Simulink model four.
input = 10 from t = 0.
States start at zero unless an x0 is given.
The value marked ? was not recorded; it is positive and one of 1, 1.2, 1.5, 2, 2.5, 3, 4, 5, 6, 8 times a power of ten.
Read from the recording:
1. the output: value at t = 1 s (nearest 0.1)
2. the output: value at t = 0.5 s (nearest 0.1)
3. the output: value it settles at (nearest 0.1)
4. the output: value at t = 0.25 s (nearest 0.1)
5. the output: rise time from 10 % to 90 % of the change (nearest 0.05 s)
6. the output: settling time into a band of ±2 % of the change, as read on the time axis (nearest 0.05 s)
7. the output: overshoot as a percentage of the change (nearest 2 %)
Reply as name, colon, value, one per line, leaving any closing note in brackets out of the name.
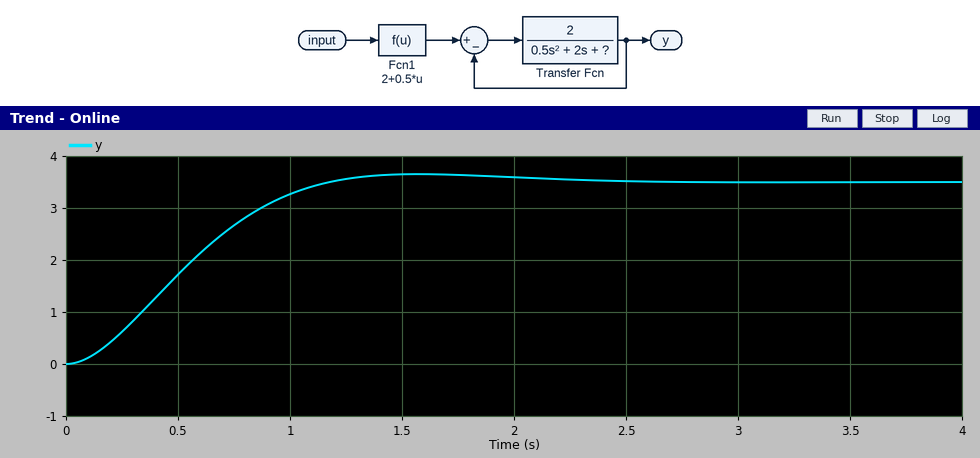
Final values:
the output: value at t = 1 s: 3.3
the output: value at t = 0.5 s: 1.7
the output: value it settles at: 3.5
the output: value at t = 0.25 s: 0.6
the output: rise time from 10 % to 90 % of the change: 0.75 s
the output: settling time into a band of ±2 % of the change, as read on the time axis: 2.10 s
the output: overshoot as a percentage of the change: 4 %
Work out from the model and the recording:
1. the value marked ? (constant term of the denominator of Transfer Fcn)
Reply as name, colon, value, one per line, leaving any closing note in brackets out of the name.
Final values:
the value marked ?: 2
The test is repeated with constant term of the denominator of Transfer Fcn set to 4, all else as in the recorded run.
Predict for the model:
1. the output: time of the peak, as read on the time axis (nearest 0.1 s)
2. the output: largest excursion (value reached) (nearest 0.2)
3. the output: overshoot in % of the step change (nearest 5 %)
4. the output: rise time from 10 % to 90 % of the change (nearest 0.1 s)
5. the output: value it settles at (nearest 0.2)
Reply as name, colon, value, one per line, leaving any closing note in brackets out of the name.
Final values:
the output: time of the peak, as read on the time axis: 1.1 s
the output: largest excursion (value reached): 2.6
the output: overshoot in % of the step change: 10 %
the output: rise time from 10 % to 90 % of the change: 0.5 s
the output: value it settles at: 2.4
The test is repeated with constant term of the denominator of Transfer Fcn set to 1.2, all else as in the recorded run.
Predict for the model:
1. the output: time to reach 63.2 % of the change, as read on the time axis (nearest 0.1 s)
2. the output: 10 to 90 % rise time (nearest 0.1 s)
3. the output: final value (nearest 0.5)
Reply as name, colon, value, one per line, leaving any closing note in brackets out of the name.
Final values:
the output: time to reach 63.2 % of the change, as read on the time axis: 0.7 s
the output: 10 to 90 % rise time: 1.0 s
the output: final value: 4.5
